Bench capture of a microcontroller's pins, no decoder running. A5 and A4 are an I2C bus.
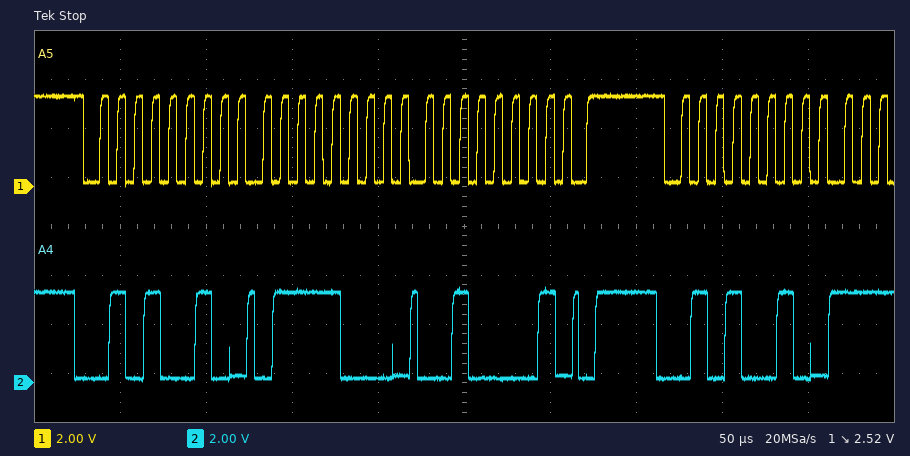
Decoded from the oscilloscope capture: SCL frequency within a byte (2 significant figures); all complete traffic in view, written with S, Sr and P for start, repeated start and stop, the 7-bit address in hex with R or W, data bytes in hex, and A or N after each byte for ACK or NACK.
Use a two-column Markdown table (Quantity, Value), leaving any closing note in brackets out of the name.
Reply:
| Quantity | Value |
|---|---|
| SCL frequency within a byte | 100 kHz |
| all complete traffic in view, written with S, Sr and P for start, repeated start and stop, the 7-bit address in hex with R or W, data bytes in hex, and A or N after each byte for ACK or NACK | S 29W A 78 A 21 A P S 29W A |
